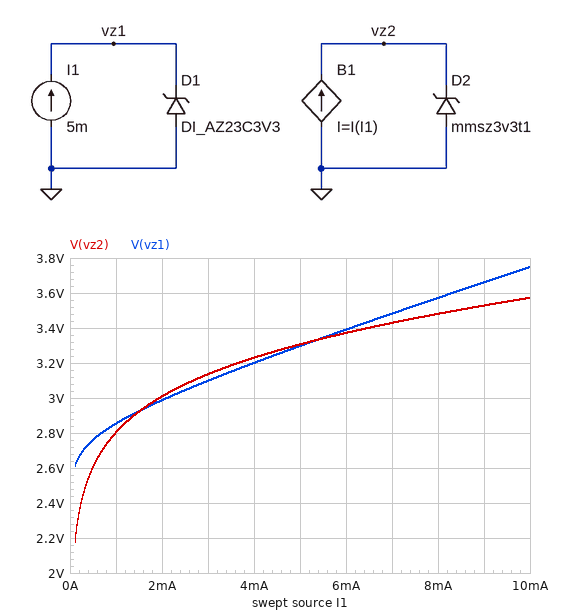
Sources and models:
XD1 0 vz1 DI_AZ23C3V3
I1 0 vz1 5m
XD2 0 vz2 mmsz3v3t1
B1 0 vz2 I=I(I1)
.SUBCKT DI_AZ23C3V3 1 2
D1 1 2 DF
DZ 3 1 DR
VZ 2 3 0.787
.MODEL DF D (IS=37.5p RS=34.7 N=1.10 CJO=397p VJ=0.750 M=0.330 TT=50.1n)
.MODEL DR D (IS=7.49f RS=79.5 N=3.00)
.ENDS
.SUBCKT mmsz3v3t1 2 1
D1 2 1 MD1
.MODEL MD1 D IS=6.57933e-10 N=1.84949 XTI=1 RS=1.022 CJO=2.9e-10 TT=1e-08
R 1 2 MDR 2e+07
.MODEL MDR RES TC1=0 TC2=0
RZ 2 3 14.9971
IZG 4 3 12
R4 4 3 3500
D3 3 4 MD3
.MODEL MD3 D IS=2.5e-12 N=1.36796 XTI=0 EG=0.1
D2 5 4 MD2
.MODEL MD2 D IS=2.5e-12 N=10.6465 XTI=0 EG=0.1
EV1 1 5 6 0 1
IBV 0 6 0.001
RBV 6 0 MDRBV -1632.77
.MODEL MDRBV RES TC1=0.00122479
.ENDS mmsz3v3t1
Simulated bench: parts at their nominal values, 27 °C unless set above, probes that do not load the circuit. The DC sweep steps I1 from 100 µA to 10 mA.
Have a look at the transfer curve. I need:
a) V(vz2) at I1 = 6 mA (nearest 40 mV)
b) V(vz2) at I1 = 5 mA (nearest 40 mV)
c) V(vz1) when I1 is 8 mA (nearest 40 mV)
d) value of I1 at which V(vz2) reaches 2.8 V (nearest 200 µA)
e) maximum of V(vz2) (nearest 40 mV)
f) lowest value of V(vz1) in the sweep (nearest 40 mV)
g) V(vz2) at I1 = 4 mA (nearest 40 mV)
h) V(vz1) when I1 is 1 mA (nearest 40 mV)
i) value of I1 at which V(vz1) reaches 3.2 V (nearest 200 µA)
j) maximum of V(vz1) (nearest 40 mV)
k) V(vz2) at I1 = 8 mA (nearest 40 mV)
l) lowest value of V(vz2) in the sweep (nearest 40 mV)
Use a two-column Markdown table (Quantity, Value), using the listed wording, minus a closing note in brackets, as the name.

| Quantity | Value |
|---|---|
| V(vz2) at I1 = 6 mA | 3.36 V |
| V(vz2) at I1 = 5 mA | 3.32 V |
| V(vz1) when I1 is 8 mA | 3.56 V |
| value of I1 at which V(vz2) reaches 2.8 V | 1.0 mA |
| maximum of V(vz2) | 3.56 V |
| lowest value of V(vz1) in the sweep | 2.60 V |
| V(vz2) at I1 = 4 mA | 3.24 V |
| V(vz1) when I1 is 1 mA | 2.84 V |
| value of I1 at which V(vz1) reaches 3.2 V | 4.0 mA |
| maximum of V(vz1) | 3.76 V |
| V(vz2) at I1 = 8 mA | 3.48 V |
| lowest value of V(vz2) in the sweep | 2.16 V |
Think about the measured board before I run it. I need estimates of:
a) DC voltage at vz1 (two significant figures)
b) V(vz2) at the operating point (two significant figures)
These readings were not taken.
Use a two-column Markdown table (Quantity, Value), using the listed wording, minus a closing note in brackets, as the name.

| Quantity | Value |
|---|---|
| DC voltage at vz1 | 3.3 V |
| V(vz2) at the operating point | 3.3 V |
